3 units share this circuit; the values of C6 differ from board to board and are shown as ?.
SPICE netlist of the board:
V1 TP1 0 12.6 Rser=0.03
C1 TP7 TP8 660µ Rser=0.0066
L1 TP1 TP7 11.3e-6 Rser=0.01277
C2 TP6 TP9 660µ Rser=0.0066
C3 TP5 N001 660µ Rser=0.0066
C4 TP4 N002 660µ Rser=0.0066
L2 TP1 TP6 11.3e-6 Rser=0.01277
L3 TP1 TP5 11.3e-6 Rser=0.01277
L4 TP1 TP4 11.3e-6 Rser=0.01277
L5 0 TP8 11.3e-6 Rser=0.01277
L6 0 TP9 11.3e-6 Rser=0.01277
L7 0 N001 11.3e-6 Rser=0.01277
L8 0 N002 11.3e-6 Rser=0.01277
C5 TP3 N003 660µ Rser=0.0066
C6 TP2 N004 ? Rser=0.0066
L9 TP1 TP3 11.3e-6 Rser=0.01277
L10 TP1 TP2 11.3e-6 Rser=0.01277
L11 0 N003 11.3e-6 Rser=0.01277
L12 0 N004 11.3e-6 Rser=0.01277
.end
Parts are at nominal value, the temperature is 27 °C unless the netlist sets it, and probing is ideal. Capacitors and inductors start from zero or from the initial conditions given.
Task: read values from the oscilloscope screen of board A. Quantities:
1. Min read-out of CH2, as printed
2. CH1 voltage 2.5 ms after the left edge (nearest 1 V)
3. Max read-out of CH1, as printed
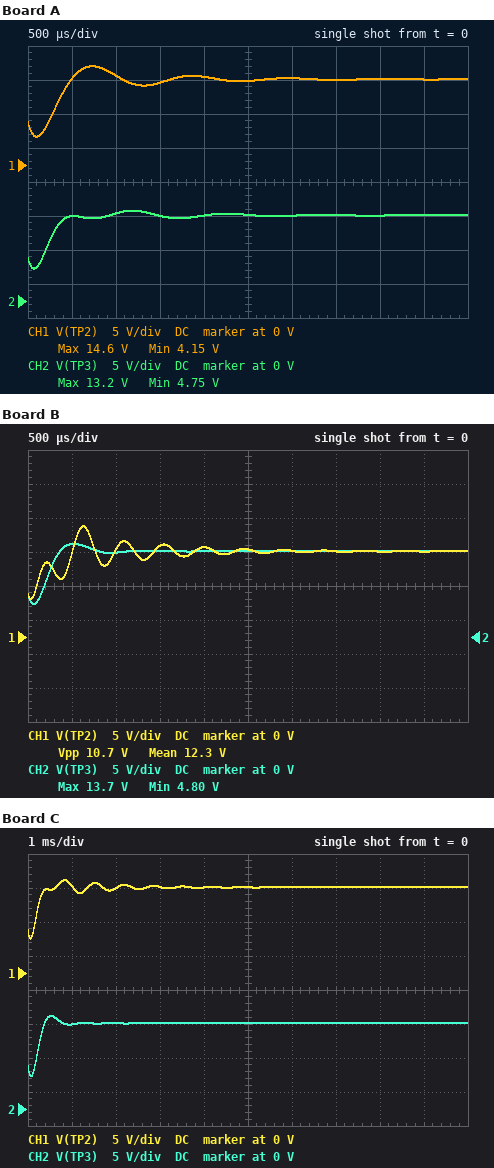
4.75 V
12 V
14.6 V
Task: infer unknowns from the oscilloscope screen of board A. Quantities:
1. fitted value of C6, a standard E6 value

1.5 mF
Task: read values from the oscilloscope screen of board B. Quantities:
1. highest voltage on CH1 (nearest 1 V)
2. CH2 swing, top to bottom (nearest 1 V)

16 V
9 V
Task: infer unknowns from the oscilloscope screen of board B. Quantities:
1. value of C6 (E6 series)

220 µF
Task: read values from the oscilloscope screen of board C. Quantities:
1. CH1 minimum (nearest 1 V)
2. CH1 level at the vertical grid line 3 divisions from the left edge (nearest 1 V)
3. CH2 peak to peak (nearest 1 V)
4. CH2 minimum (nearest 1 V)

5 V
13 V
9 V
5 V
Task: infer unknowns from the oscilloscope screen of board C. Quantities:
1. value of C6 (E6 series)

470 µF
